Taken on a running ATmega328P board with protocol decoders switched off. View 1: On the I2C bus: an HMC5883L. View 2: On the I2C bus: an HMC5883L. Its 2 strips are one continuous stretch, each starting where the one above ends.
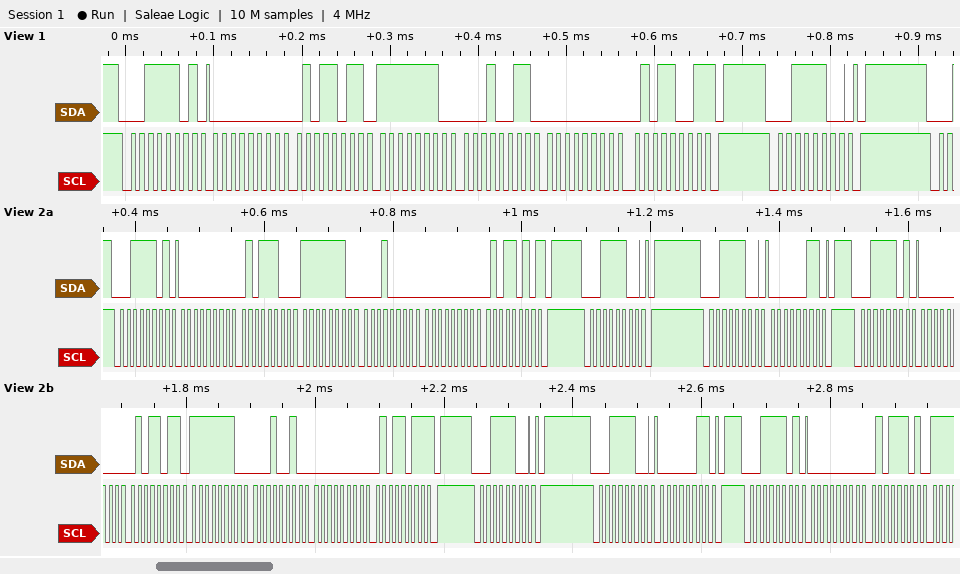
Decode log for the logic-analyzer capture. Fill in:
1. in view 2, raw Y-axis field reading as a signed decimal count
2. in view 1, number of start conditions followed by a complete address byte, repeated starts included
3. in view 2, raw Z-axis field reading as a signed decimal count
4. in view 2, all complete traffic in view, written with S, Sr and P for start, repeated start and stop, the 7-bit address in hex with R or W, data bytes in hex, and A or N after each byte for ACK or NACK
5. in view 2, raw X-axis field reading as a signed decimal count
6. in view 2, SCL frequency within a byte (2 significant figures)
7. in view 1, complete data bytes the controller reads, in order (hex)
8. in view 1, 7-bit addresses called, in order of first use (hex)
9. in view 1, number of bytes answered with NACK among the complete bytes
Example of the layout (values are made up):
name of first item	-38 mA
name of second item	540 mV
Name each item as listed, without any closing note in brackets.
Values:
in view 2, raw Y-axis field reading as a signed decimal count	91
in view 1, number of start conditions followed by a complete address byte, repeated starts included	2
in view 2, raw Z-axis field reading as a signed decimal count	-494
in view 2, all complete traffic in view, written with S, Sr and P for start, repeated start and stop, the 7-bit address in hex with R or W, data bytes in hex, and A or N after each byte for ACK or NACK	S 1ER A 00 A 5C A FE A 10 A 00 A 5A N P S 1EW A P S 1EW A 03 A P S 1ER A 00 A 5B A FE A 12 A 00 A 5B N P S 1EW A P S 1EW A 03 A P S 1ER A 00 A 5D A
in view 2, raw X-axis field reading as a signed decimal count	91
in view 2, SCL frequency within a byte	100 kHz
in view 1, complete data bytes the controller reads, in order	00 5B FE 13 00 59
in view 1, 7-bit addresses called, in order of first use	0x1E
in view 1, number of bytes answered with NACK among the complete bytes	1
